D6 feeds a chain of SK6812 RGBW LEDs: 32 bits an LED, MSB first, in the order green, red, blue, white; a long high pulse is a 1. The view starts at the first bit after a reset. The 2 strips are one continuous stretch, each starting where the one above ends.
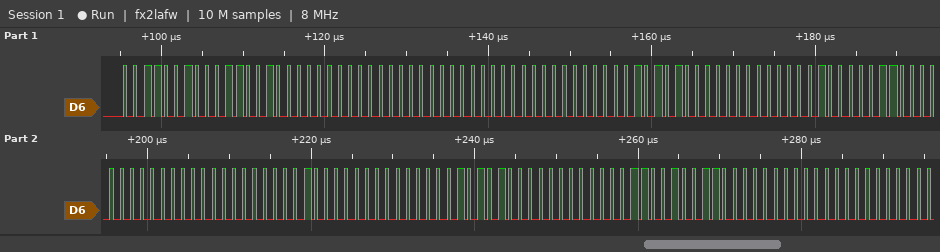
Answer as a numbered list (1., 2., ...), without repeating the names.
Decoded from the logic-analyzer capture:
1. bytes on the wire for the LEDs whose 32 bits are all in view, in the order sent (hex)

1. 32 32 00 00 00 00 2A 00 08 30 00 00 10 00 2A 00 19 30 00 00
